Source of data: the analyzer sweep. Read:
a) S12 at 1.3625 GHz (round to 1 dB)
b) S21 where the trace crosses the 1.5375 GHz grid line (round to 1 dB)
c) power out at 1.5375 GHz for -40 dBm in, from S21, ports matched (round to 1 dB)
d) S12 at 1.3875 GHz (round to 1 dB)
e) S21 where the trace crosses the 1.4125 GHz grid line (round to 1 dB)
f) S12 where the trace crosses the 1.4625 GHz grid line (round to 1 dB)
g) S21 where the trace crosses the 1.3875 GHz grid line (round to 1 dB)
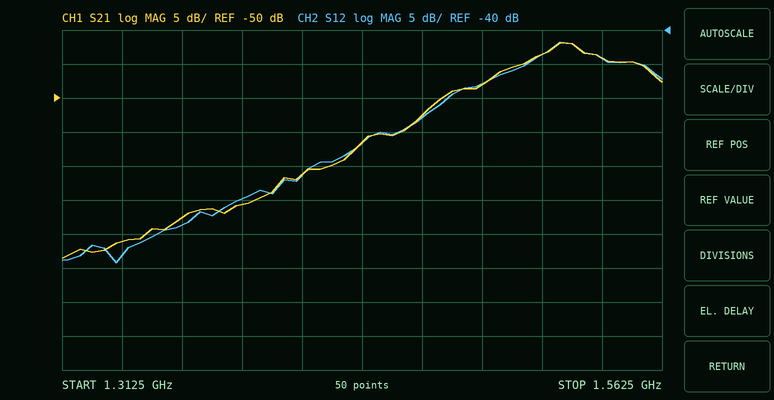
-69 dB
-44 dB
-84 dBm
-65 dB
-61 dB
-53 dB
-66 dB
